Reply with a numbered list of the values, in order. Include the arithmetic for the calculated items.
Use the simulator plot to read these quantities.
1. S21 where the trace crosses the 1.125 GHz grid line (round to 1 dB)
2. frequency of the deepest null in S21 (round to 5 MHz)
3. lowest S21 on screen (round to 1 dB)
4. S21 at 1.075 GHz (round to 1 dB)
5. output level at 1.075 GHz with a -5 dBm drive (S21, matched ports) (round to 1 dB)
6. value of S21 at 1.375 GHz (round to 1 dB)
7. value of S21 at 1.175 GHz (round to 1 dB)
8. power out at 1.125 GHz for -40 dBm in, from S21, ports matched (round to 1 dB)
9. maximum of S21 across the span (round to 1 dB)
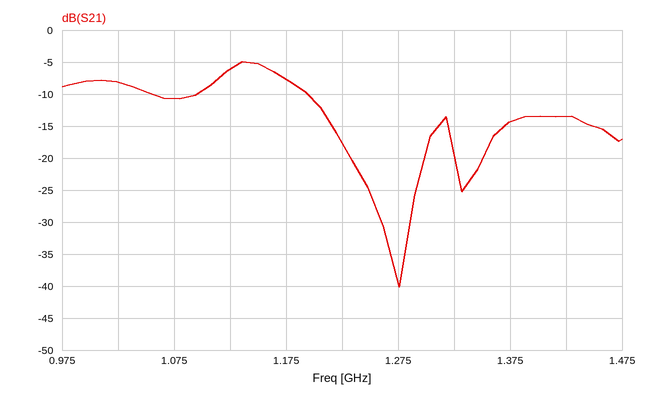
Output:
1. -6 dB
2. 1.275 GHz
3. -40 dB
4. -11 dB
5. -5 dBm + (-11 dB) = -16 dBm
6. -14 dB
7. -8 dB
8. -40 dBm + (-6 dB) = -46 dBm
9. -5 dB
